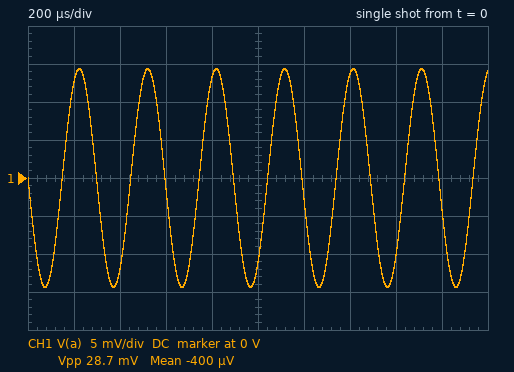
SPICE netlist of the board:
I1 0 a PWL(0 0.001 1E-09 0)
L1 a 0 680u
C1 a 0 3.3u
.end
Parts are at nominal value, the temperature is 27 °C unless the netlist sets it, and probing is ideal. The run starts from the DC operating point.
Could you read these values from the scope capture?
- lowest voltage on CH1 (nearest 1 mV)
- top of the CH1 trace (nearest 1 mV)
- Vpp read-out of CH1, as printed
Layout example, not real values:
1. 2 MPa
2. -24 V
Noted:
1. -14 mV
2. 14 mV
3. 28.7 mV
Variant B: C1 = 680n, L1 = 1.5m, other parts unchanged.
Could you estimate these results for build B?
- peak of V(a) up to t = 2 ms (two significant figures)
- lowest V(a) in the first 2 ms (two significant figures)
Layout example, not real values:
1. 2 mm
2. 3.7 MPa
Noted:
1. 47 mV
2. -47 mV
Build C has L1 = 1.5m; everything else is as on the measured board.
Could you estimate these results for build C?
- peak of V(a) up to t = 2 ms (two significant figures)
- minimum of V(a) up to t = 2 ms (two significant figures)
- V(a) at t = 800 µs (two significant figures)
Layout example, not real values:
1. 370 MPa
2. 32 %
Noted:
1. 21 mV
2. -21 mV
3. 20 mV
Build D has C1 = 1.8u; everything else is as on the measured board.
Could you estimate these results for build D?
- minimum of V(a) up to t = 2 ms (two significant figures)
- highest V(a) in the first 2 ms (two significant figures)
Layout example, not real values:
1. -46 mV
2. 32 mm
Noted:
1. -19 mV
2. 19 mV
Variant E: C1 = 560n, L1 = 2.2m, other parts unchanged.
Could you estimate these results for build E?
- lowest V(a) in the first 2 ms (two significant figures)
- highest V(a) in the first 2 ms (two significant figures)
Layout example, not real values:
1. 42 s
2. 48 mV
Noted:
1. -63 mV
2. 63 mV
